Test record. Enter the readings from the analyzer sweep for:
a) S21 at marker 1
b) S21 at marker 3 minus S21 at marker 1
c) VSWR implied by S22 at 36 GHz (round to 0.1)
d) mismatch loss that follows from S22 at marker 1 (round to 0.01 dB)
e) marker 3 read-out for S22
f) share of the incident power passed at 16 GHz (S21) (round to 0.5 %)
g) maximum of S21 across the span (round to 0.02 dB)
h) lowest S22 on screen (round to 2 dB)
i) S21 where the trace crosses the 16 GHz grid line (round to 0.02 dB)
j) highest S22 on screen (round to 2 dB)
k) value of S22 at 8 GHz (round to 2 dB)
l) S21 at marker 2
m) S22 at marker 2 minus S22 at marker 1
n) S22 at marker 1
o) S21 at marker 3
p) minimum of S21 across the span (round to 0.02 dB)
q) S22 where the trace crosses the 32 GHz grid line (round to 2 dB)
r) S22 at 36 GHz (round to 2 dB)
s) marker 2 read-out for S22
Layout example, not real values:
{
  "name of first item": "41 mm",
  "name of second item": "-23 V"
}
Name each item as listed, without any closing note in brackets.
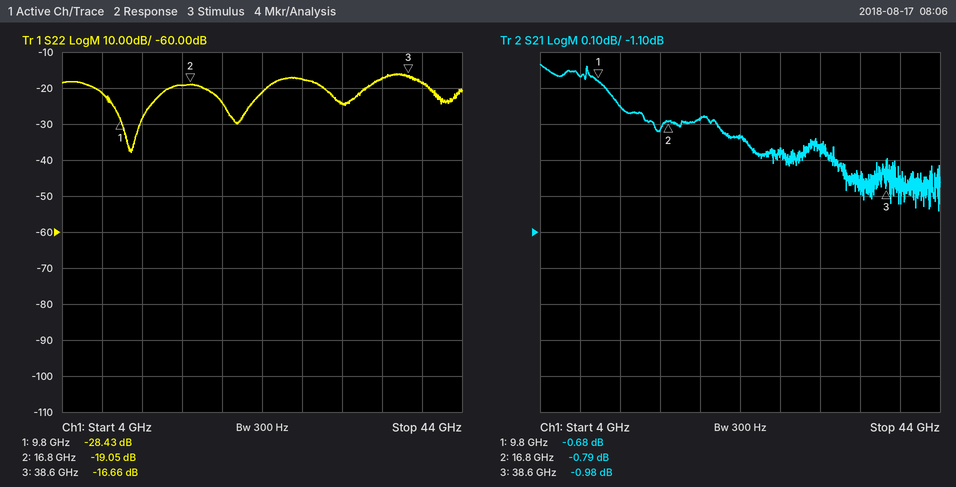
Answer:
{
  "S21 at marker 1": "-0.68 dB",
  "S21 at marker 3 minus S21 at marker 1": "-0.30 dB",
  "VSWR implied by S22 at 36 GHz": "1.3",
  "mismatch loss that follows from S22 at marker 1": "0.01 dB",
  "marker 3 read-out for S22": "-16.66 dB",
  "share of the incident power passed at 16 GHz (S21)": "83.0 %",
  "maximum of S21 across the span": "-0.64 dB",
  "lowest S22 on screen": "-38 dB",
  "S21 where the trace crosses the 16 GHz grid line": "-0.82 dB",
  "highest S22 on screen": "-16 dB",
  "value of S22 at 8 GHz": "-22 dB",
  "S21 at marker 2": "-0.79 dB",
  "S22 at marker 2 minus S22 at marker 1": "9.38 dB",
  "S22 at marker 1": "-28.43 dB",
  "S21 at marker 3": "-0.98 dB",
  "minimum of S21 across the span": "-1.04 dB",
  "S22 where the trace crosses the 32 GHz grid line": "-24 dB",
  "S22 at 36 GHz": "-18 dB",
  "marker 2 read-out for S22": "-19.05 dB"
}
